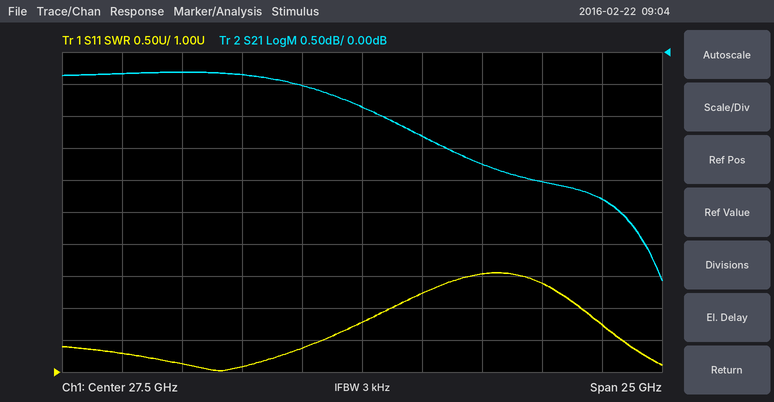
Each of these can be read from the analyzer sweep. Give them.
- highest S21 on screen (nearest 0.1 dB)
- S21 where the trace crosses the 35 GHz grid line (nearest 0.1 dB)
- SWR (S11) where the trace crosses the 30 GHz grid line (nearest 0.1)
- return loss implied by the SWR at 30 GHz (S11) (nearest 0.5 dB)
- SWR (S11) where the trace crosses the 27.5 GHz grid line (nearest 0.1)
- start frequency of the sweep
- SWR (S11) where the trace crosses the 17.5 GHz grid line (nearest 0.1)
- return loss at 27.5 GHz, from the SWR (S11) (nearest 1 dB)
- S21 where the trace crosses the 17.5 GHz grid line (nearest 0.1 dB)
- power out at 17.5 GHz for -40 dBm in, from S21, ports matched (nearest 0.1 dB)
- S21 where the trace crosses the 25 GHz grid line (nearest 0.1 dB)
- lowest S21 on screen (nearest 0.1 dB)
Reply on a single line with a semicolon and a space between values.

-0.3 dB; -2.0 dB; 2.2; 8.5 dB; 1.8; 15 GHz; 1.3; 11 dB; -0.3 dB; -40.3 dBm; -0.5 dB; -3.6 dB
